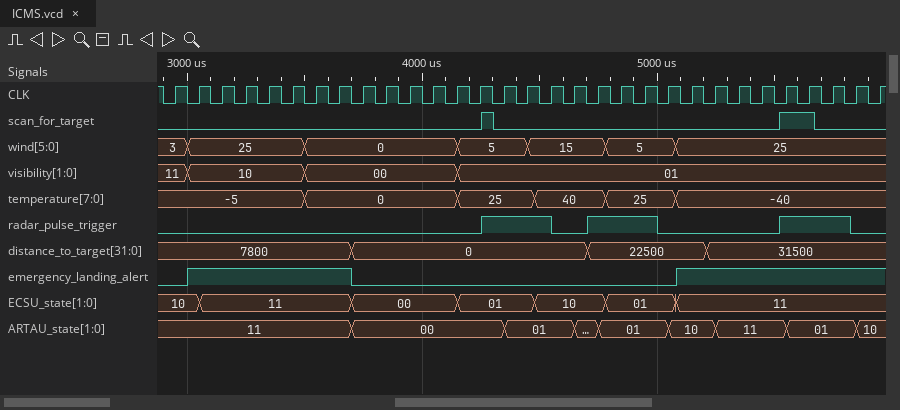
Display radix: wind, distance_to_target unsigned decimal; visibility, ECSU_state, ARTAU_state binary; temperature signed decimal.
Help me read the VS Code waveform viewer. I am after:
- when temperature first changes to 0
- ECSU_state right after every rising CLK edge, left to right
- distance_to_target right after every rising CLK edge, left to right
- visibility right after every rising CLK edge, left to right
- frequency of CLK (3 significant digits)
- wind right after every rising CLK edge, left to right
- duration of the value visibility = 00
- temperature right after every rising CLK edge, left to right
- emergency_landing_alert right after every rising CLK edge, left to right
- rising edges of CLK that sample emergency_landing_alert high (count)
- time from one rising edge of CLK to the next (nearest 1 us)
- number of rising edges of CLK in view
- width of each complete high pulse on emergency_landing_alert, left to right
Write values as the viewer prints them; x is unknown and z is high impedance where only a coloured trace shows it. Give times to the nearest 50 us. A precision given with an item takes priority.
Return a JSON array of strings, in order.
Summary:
["3500 us", "10, 11, 11, 11, 11, 11, 11, 11, 00, 00, 00, 00, 01, 01, 01, 01, 10, 10, 10, 01, 01, 01, 11, 11, 11, 11, 11, 11, 11, 11, 11", "7800, 7800, 7800, 7800, 7800, 7800, 7800, 7800, 0, 0, 0, 0, 0, 0, 0, 0, 0, 0, 22500, 22500, 22500, 22500, 22500, 31500, 31500, 31500, 31500, 31500, 31500, 31500, 31500", "11, 10, 10, 10, 10, 10, 00, 00, 00, 00, 00, 00, 01, 01, 01, 01, 01, 01, 01, 01, 01, 01, 01, 01, 01, 01, 01, 01, 01, 01, 01", "10.0 kHz", "3, 25, 25, 25, 25, 25, 0, 0, 0, 0, 0, 0, 5, 5, 5, 15, 15, 15, 15, 5, 5, 5, 25, 25, 25, 25, 25, 25, 25, 25, 25", "650 us", "-5, -5, -5, -5, -5, -5, 0, 0, 0, 0, 0, 0, 25, 25, 25, 25, 40, 40, 40, 25, 25, 25, -40, -40, -40, -40, -40, -40, -40, -40, -40", "0 1 1 1 1 1 1 1 0 0 0 0 0 0 0 0 0 0 0 0 0 0 1 1 1 1 1 1 1 1 1", "16", "100 us", "31", "700 us"]
